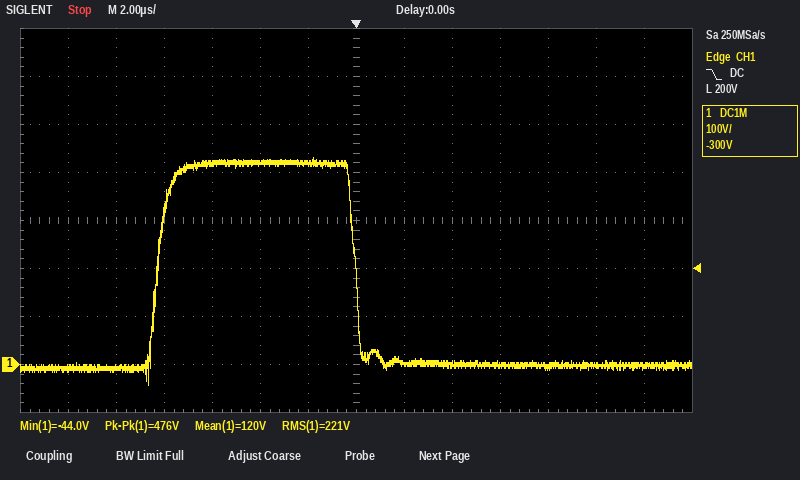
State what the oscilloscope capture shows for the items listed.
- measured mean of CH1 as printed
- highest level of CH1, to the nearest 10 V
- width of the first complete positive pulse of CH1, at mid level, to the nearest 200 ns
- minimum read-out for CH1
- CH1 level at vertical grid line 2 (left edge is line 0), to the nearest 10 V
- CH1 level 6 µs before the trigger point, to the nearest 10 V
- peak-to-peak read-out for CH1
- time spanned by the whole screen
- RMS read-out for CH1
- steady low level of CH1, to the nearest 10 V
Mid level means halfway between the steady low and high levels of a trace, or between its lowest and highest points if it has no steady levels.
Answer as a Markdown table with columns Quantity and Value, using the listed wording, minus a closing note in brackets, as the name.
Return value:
| Quantity | Value |
|---|---|
| measured mean of CH1 as printed | 120 V |
| highest level of CH1, to the nearest 10 V | 430 V |
| width of the first complete positive pulse of CH1, at mid level, to the nearest 200 ns | 8.2 µs |
| minimum read-out for CH1 | -44.0 V |
| CH1 level at vertical grid line 2 (left edge is line 0), to the nearest 10 V | -10 V |
| CH1 level 6 µs before the trigger point, to the nearest 10 V | 420 V |
| peak-to-peak read-out for CH1 | 476 V |
| time spanned by the whole screen | 28 µs |
| RMS read-out for CH1 | 221 V |
| steady low level of CH1, to the nearest 10 V | 0 V |
